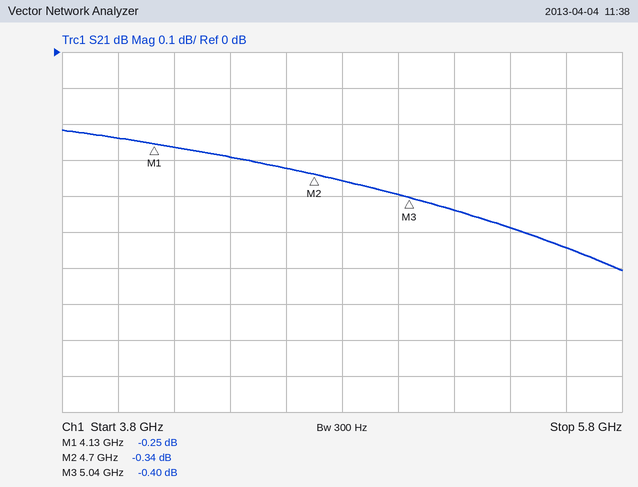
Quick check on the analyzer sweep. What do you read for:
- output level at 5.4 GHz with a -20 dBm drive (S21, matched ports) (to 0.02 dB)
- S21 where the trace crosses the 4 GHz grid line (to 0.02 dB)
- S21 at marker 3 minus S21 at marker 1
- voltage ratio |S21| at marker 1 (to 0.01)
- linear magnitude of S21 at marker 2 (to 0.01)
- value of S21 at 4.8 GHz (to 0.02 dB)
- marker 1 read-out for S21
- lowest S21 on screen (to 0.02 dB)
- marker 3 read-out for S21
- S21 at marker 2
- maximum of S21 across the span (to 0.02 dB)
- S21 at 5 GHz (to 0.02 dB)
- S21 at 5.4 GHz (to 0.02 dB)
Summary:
-20.48 dBm
-0.24 dB
-0.15 dB
0.97
0.96
-0.36 dB
-0.25 dB
-0.60 dB
-0.40 dB
-0.34 dB
-0.22 dB
-0.40 dB
-0.48 dB
